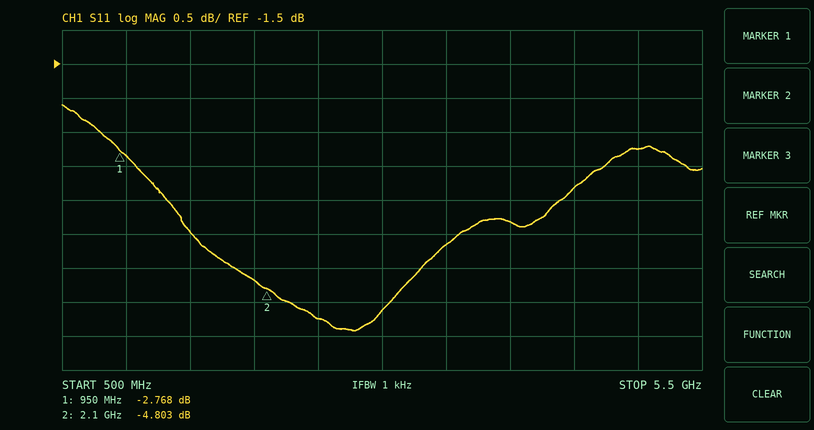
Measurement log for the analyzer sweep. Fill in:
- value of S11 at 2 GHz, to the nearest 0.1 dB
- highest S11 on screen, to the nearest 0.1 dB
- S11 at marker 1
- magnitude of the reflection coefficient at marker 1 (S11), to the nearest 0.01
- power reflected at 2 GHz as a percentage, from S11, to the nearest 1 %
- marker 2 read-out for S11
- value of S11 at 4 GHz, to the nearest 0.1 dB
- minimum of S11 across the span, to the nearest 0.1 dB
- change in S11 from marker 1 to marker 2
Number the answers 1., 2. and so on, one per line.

1. -4.7 dB
2. -2.1 dB
3. -2.768 dB
4. 0.73
5. 34 %
6. -4.803 dB
7. -3.8 dB
8. -5.4 dB
9. -2.035 dB
